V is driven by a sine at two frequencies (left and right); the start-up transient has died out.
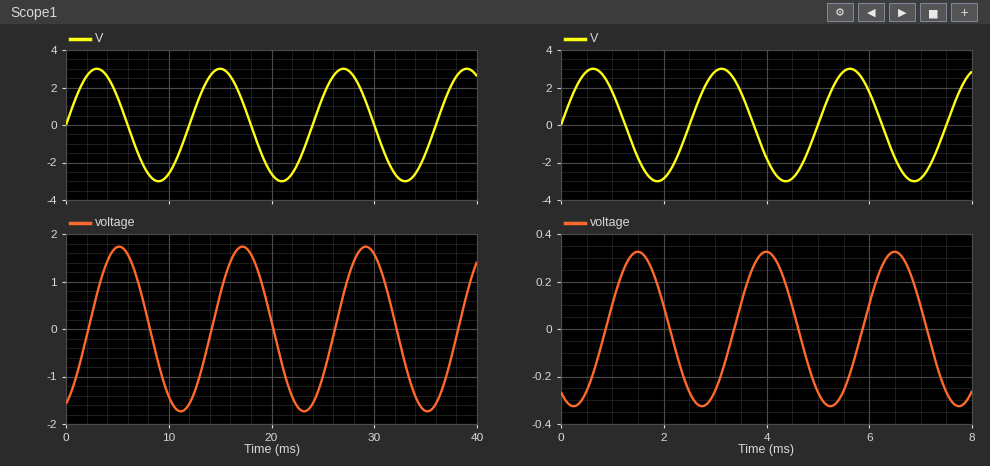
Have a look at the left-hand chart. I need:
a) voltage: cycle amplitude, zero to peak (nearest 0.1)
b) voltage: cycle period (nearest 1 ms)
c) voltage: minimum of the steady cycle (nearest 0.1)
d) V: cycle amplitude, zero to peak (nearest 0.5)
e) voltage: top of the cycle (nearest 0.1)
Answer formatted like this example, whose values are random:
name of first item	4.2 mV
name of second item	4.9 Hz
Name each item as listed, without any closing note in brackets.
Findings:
voltage: cycle amplitude, zero to peak	1.7
voltage: cycle period	12 ms
voltage: minimum of the steady cycle	-1.7
V: cycle amplitude, zero to peak	3.0
voltage: top of the cycle	1.7
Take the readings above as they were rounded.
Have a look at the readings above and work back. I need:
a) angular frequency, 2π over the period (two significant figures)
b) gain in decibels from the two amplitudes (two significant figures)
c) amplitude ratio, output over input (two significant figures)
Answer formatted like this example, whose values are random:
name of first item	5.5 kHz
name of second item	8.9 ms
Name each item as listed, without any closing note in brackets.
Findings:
angular frequency, 2π over the period	0.52 rad/ms
gain in decibels from the two amplitudes	-4.9 dB
amplitude ratio, output over input	0.57
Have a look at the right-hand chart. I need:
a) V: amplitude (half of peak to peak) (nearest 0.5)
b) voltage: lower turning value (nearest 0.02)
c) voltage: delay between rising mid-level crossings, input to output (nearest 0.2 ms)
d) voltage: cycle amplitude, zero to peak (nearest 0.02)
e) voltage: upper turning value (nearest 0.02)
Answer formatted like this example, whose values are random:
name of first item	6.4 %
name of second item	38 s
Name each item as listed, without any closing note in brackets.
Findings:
V: amplitude (half of peak to peak)	3.0
voltage: lower turning value	-0.32
voltage: delay between rising mid-level crossings, input to output	0.8 ms
voltage: cycle amplitude, zero to peak	0.32
voltage: upper turning value	0.32
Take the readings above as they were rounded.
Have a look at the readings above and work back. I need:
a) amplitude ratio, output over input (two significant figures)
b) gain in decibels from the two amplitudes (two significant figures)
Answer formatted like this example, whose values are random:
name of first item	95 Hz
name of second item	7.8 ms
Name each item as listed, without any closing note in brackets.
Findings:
amplitude ratio, output over input	0.11
gain in decibels from the two amplitudes	-19 dB
